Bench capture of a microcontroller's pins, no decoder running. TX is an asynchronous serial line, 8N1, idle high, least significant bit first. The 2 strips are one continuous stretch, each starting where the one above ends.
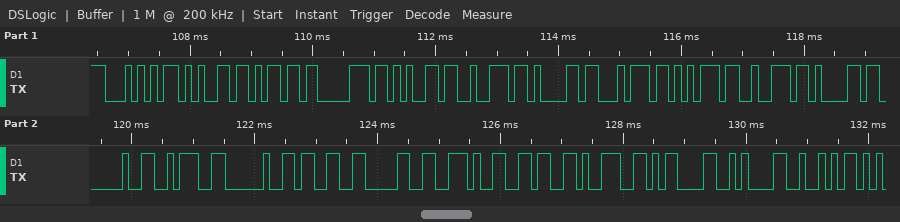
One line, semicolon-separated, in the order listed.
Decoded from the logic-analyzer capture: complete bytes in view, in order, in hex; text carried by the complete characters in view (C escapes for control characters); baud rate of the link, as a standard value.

54 65 6D 70 65 72 61 74 75 72 61 20 3A 20 33 30 2E 36 39 0D 0A 52; "Temperatura : 30.69\r\nR"; 9600 baud
